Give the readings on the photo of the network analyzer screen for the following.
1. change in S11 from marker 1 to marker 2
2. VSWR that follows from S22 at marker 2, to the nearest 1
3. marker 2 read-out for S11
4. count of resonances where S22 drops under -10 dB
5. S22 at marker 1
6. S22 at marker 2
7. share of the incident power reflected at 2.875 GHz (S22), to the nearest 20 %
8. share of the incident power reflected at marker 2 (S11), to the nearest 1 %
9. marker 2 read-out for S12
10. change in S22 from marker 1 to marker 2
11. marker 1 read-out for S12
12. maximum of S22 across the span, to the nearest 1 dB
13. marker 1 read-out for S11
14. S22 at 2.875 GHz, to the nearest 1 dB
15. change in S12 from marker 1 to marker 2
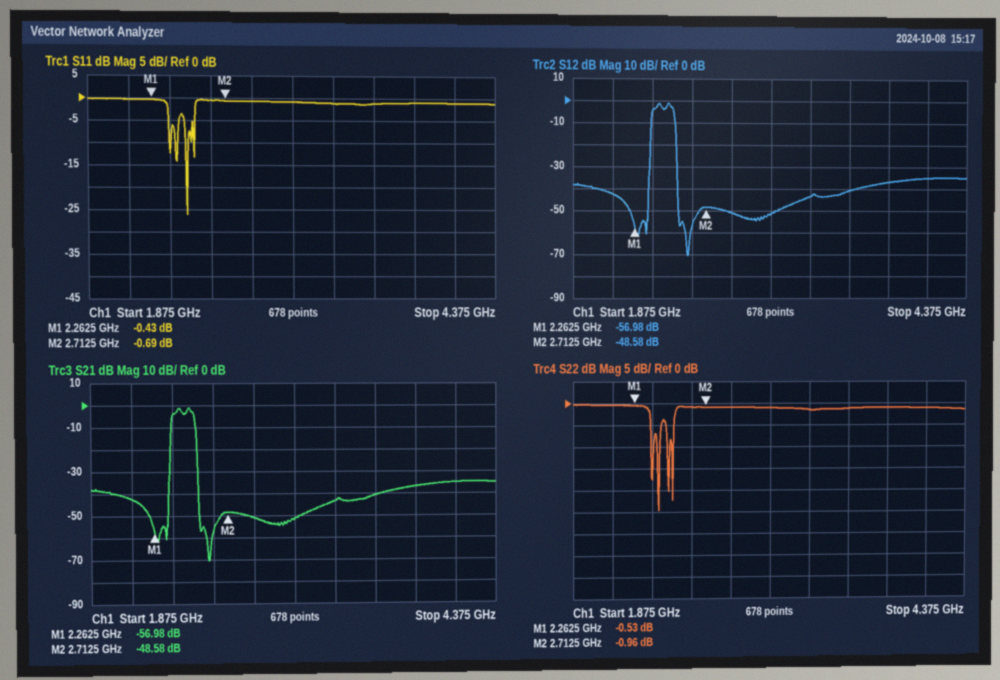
-0.26 dB
18
-0.69 dB
4
-0.53 dB
-0.96 dB
80 %
85 %
-48.58 dB
-0.43 dB
-56.98 dB
0 dB
-0.43 dB
-1 dB
8.40 dB
